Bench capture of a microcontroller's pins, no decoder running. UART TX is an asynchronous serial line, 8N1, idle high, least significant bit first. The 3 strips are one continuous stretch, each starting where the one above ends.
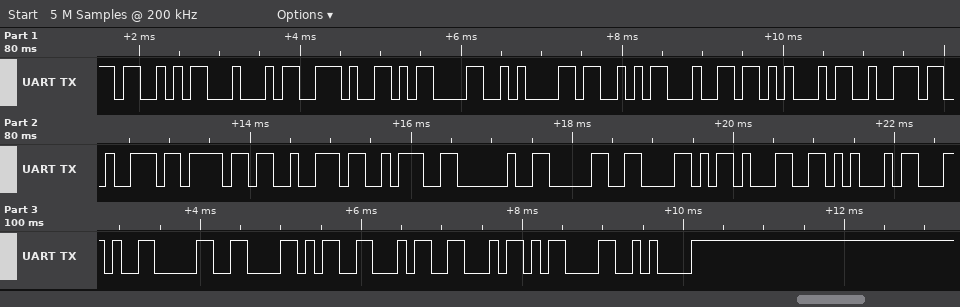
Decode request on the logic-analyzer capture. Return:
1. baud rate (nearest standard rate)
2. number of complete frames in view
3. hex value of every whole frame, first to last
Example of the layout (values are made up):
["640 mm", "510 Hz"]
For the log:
["9600 baud", "25", "53 44 2E 0D 0A 53 64 45 72 72 6F 72 3A 20 30 58 31 45 2C 30 58 46 46 0D 0A"]
